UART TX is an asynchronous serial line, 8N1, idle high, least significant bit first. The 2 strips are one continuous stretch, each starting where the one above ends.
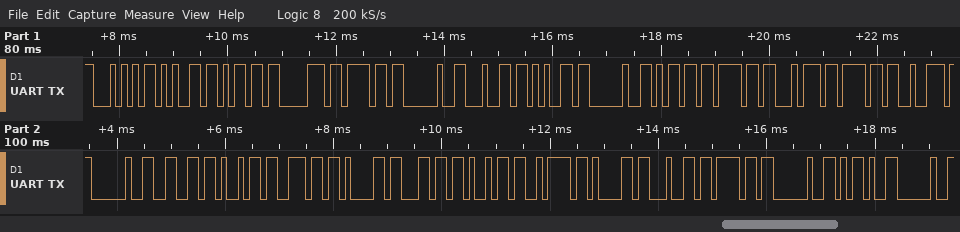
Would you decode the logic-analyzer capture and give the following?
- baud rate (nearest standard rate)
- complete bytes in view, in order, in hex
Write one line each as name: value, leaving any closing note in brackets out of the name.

baud rate: 9600 baud
complete bytes in view, in order, in hex: 0x54 0x65 0x6D 0x70 0x6F 0x20 0x64 0x65 0x20 0x6D 0x6F 0x74 0x6F 0x72 0x20 0x66 0x69 0x6E 0x61 0x6C 0x69 0x7A 0x61 0x64 0x6F 0x20 0x2D 0x20
